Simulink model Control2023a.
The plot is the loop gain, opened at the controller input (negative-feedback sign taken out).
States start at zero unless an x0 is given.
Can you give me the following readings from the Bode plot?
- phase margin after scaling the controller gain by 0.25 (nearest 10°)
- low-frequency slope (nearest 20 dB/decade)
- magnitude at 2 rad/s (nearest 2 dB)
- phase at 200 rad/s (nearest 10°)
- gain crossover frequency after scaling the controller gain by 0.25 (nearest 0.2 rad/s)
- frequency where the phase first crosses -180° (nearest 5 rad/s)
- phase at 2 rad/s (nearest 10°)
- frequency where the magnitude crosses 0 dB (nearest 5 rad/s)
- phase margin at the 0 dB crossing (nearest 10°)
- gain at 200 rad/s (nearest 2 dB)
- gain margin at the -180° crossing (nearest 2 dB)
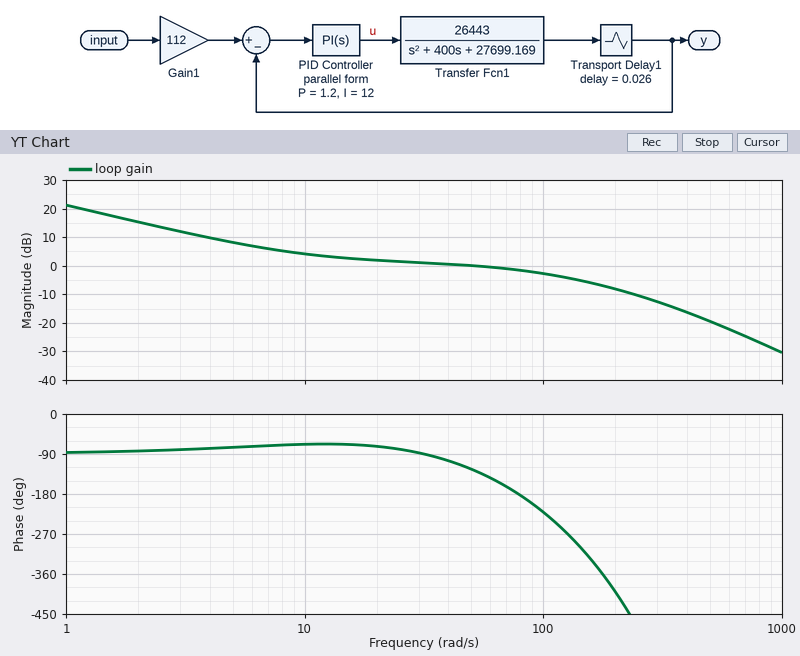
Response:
100°
-20 dB/decade
16 dB
-400°
3.0 rad/s
80 rad/s
-80°
50 rad/s
50°
-8 dB
2 dB
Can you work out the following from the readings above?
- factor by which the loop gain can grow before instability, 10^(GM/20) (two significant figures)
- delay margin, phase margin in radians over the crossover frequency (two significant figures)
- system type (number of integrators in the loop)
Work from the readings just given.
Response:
1.3
0.017 s
1
